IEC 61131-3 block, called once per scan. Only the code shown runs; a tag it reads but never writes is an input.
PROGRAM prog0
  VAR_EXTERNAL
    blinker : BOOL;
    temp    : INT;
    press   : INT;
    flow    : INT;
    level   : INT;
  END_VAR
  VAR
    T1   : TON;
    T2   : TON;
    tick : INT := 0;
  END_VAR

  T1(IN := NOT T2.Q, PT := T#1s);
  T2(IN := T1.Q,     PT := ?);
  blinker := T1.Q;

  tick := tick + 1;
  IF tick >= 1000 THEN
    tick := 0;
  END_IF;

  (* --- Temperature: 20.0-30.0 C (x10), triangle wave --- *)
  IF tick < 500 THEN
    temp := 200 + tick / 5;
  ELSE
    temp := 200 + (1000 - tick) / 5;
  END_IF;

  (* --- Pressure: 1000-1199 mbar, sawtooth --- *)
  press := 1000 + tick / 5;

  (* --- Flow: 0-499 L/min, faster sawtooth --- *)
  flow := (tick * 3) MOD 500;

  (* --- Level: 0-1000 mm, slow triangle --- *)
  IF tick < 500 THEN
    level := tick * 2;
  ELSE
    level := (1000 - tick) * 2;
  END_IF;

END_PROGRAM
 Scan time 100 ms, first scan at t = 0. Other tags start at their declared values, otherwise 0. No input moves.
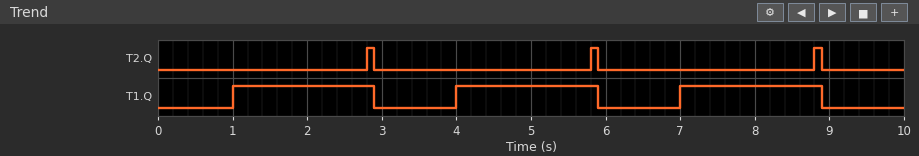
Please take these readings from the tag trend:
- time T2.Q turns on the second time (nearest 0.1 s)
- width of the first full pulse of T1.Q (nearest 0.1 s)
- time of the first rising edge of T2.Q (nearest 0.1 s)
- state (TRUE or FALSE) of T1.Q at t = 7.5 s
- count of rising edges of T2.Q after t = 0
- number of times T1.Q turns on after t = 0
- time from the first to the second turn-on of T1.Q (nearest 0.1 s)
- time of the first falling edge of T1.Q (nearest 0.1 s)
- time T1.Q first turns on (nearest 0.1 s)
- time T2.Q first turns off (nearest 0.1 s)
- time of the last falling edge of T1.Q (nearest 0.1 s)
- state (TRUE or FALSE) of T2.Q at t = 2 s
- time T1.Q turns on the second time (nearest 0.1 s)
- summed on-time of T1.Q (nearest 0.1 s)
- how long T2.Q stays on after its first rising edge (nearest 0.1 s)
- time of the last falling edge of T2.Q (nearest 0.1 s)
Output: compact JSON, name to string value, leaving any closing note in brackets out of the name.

{"time T2.Q turns on the second time": "5.8 s", "width of the first full pulse of T1.Q": "1.9 s", "time of the first rising edge of T2.Q": "2.8 s", "state (TRUE or FALSE) of T1.Q at t = 7.5 s": "TRUE", "count of rising edges of T2.Q after t = 0": "3", "number of times T1.Q turns on after t = 0": "3", "time from the first to the second turn-on of T1.Q": "3.0 s", "time of the first falling edge of T1.Q": "2.9 s", "time T1.Q first turns on": "1.0 s", "time T2.Q first turns off": "2.9 s", "time of the last falling edge of T1.Q": "8.9 s", "state (TRUE or FALSE) of T2.Q at t = 2 s": "FALSE", "time T1.Q turns on the second time": "4.0 s", "summed on-time of T1.Q": "5.7 s", "how long T2.Q stays on after its first rising edge": "0.1 s", "time of the last falling edge of T2.Q": "8.9 s"}
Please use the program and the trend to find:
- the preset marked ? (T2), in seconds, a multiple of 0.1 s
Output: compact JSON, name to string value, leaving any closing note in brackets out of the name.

{"the preset marked ? (T2), in seconds, a multiple of 0.1 s": "1.8 s"}
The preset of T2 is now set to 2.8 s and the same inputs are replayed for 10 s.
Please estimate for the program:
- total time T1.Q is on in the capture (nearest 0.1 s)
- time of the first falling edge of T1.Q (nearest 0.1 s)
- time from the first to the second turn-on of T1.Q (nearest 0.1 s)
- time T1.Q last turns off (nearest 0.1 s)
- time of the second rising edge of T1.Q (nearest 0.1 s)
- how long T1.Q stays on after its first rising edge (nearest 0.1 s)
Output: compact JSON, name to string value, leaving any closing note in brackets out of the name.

{"total time T1.Q is on in the capture": "6.8 s", "time of the first falling edge of T1.Q": "3.9 s", "time from the first to the second turn-on of T1.Q": "4.0 s", "time T1.Q last turns off": "7.9 s", "time of the second rising edge of T1.Q": "5.0 s", "how long T1.Q stays on after its first rising edge": "2.9 s"}
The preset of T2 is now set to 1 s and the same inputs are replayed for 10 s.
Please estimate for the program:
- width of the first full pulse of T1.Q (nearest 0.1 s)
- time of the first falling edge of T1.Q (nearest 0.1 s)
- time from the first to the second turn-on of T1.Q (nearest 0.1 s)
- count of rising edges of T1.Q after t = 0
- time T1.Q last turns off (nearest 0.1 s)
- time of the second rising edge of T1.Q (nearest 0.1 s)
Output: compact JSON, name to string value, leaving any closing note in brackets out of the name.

{"width of the first full pulse of T1.Q": "1.1 s", "time of the first falling edge of T1.Q": "2.1 s", "time from the first to the second turn-on of T1.Q": "2.2 s", "count of rising edges of T1.Q after t = 0": "5", "time T1.Q last turns off": "8.7 s", "time of the second rising edge of T1.Q": "3.2 s"}
